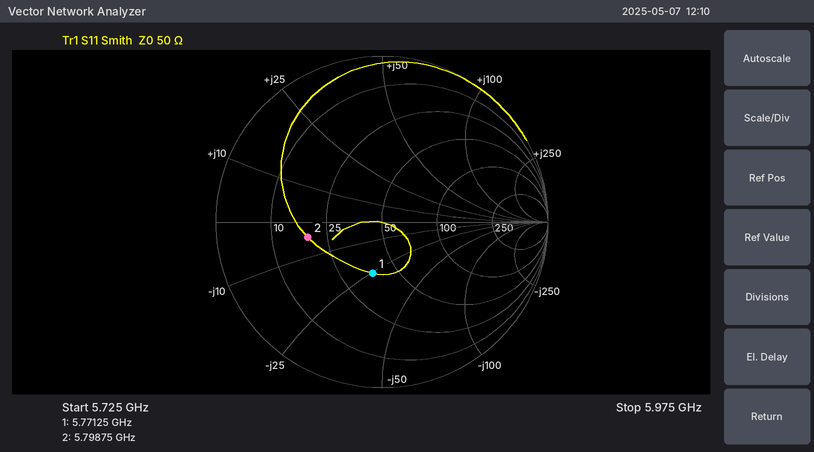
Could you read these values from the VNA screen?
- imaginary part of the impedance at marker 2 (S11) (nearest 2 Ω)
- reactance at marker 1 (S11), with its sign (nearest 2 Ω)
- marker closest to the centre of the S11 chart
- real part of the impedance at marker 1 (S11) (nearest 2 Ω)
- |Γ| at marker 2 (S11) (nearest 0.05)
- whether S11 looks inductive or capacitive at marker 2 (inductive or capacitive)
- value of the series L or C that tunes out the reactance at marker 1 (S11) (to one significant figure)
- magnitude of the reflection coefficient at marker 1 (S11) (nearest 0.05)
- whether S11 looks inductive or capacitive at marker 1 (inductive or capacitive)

-4 Ω
-26 Ω
marker 1
38 Ω
0.45
capacitive
700 pH
0.30
capacitive
